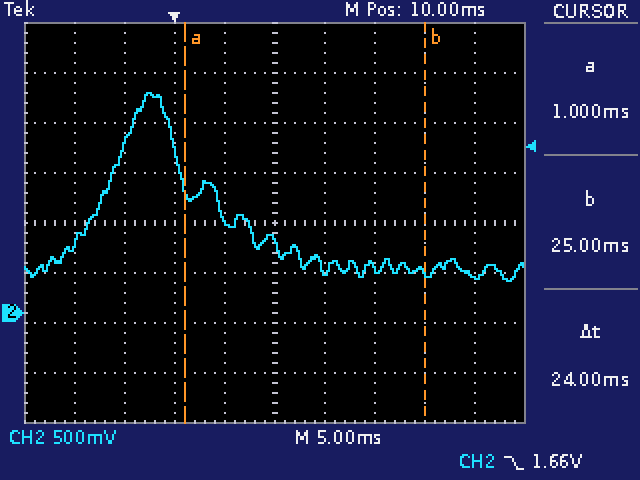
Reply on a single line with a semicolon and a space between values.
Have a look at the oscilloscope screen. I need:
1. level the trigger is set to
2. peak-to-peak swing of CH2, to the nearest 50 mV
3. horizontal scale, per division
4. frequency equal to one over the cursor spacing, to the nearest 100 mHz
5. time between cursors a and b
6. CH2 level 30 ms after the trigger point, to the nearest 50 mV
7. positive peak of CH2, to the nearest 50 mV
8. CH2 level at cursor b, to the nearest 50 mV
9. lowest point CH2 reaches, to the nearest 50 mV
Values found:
1.66 V; 1.90 V; 5 ms; 41.7 Hz; 24 ms; 350 mV; 2.20 V; 400 mV; 300 mV
